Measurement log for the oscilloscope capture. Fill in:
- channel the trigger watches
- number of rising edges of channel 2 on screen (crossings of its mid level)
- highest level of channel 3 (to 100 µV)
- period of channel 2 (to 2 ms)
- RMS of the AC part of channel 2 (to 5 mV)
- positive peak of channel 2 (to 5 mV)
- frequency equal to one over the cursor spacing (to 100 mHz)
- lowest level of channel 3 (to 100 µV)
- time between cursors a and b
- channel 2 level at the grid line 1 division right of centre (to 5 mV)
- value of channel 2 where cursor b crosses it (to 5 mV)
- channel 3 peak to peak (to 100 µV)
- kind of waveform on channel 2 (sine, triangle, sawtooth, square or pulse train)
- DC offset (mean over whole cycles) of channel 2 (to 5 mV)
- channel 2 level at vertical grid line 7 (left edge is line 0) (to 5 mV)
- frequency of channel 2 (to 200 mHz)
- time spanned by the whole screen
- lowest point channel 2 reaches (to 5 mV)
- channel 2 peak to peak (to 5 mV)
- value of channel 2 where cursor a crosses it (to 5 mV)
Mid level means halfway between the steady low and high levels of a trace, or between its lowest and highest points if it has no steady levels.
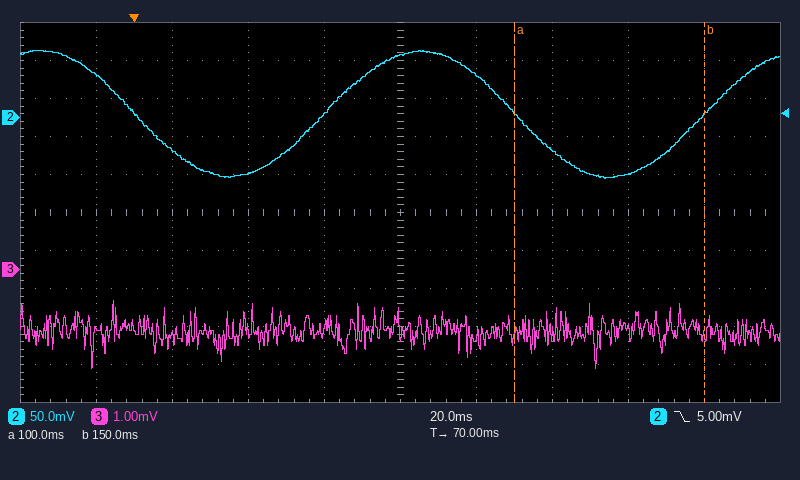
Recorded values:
channel 2
2
-800 µV
100 ms
60 mV
90 mV
20.0 Hz
-2.6 mV
50 ms
55 mV
5 mV
1.8 mV
sine
5 mV
-45 mV
10.0 Hz
200 ms
-80 mV
170 mV
5 mV
